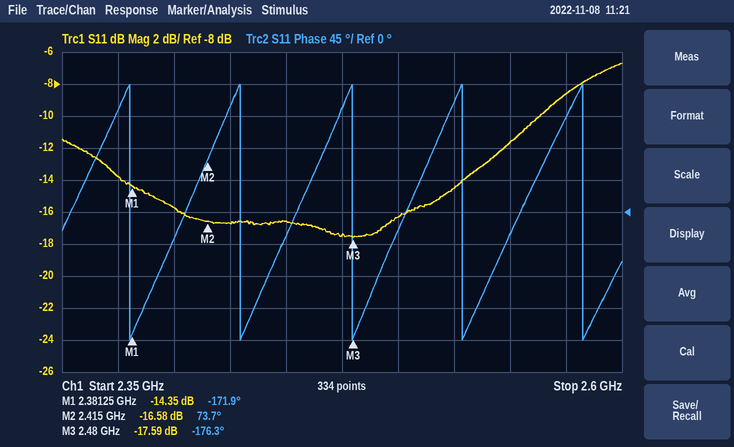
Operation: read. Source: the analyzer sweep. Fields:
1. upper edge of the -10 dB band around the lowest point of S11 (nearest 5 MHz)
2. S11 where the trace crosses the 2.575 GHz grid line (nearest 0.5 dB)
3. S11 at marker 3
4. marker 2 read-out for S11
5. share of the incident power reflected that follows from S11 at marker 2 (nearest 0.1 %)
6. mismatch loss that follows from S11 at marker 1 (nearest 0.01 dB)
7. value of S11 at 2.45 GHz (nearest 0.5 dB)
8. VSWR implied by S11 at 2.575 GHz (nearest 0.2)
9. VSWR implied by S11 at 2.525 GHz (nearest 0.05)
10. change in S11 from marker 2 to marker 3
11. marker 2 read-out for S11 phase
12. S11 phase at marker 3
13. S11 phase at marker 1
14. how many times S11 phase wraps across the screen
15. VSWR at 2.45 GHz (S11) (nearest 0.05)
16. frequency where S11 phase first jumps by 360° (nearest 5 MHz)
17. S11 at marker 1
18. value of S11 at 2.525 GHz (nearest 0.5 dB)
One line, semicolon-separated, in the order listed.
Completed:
2.565 GHz; -8.5 dB; -17.59 dB; -16.58 dB; 2.2 %; 0.16 dB; -16.5 dB; 2.2; 1.45; -1.01 dB; 73.7°; -176.3°; -171.9°; 5; 1.35; 2.380 GHz; -14.35 dB; -14.5 dB
